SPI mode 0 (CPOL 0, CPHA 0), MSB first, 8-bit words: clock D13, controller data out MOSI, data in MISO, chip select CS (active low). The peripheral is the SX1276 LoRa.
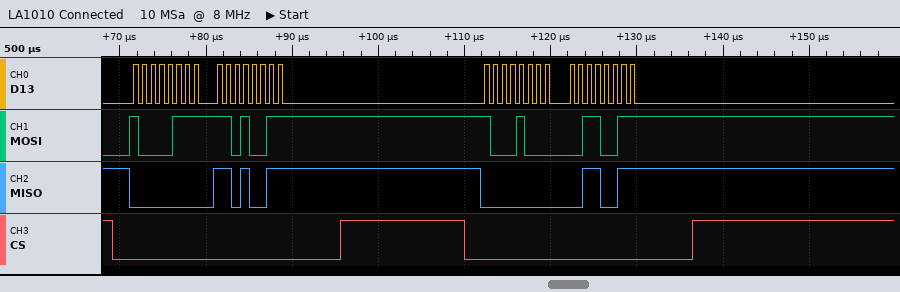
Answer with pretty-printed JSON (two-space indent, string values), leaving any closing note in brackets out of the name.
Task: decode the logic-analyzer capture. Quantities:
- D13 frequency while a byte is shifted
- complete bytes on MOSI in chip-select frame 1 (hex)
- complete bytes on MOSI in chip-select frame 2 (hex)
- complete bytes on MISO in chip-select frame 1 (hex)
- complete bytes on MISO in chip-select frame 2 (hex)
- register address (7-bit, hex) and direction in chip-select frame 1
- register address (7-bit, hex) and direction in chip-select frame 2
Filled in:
{
  "D13 frequency while a byte is shifted": "1 MHz",
  "complete bytes on MOSI in chip-select frame 1": "0x87 0xD3",
  "complete bytes on MOSI in chip-select frame 2": "0x88 0x33",
  "complete bytes on MISO in chip-select frame 1": "0x00 0xD3",
  "complete bytes on MISO in chip-select frame 2": "0x00 0x33",
  "register address (7-bit, hex) and direction in chip-select frame 1": "0x07 write",
  "register address (7-bit, hex) and direction in chip-select frame 2": "0x08 write"
}
